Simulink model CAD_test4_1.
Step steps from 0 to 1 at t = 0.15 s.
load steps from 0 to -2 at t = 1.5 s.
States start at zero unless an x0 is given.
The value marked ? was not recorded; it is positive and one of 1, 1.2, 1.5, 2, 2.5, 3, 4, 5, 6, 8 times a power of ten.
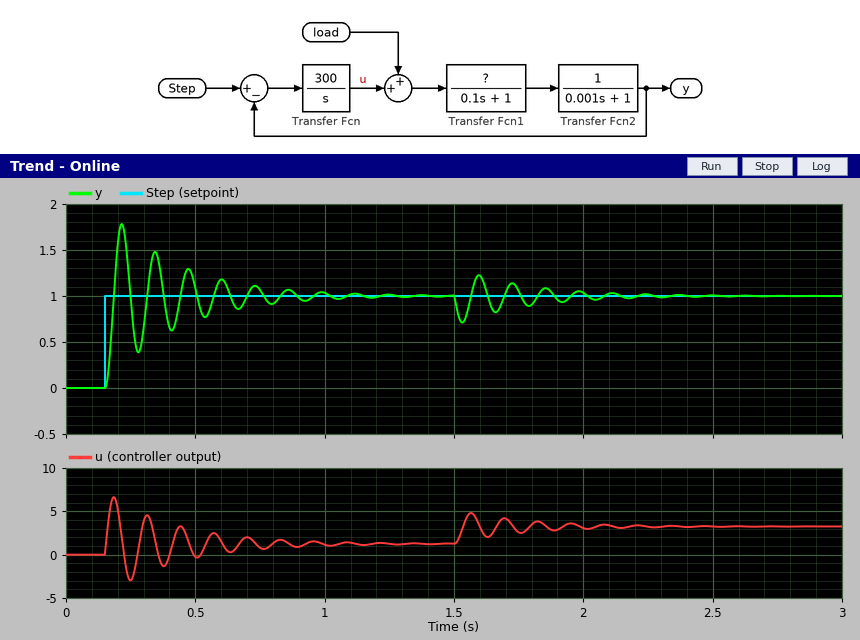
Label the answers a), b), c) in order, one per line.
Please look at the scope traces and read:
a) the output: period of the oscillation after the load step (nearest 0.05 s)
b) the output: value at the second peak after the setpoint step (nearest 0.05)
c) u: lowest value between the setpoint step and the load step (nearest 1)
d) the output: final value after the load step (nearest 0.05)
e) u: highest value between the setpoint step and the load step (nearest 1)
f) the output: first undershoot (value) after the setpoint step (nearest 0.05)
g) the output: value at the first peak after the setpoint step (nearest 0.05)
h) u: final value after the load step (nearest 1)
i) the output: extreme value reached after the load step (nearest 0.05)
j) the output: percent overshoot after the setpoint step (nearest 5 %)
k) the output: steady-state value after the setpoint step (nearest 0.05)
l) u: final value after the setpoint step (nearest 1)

a) 0.15 s
b) 1.50
c) -3
d) 1.00
e) 7
f) 0.40
g) 1.80
h) 3
i) 0.70
j) 80 %
k) 1.00
l) 1
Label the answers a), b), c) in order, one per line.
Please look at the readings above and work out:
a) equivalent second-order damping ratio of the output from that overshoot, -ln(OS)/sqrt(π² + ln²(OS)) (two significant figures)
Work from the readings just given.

a) 0.071
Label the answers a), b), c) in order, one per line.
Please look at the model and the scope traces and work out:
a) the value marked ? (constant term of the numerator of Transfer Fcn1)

a) 0.8
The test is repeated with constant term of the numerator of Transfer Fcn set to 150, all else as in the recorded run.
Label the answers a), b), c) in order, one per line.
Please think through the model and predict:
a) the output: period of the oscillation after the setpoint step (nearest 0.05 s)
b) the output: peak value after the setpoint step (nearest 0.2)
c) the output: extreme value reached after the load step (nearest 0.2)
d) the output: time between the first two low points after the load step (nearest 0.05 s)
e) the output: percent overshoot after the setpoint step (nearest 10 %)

a) 0.20 s
b) 1.6
c) 0.6
d) 0.20 s
e) 70 %
